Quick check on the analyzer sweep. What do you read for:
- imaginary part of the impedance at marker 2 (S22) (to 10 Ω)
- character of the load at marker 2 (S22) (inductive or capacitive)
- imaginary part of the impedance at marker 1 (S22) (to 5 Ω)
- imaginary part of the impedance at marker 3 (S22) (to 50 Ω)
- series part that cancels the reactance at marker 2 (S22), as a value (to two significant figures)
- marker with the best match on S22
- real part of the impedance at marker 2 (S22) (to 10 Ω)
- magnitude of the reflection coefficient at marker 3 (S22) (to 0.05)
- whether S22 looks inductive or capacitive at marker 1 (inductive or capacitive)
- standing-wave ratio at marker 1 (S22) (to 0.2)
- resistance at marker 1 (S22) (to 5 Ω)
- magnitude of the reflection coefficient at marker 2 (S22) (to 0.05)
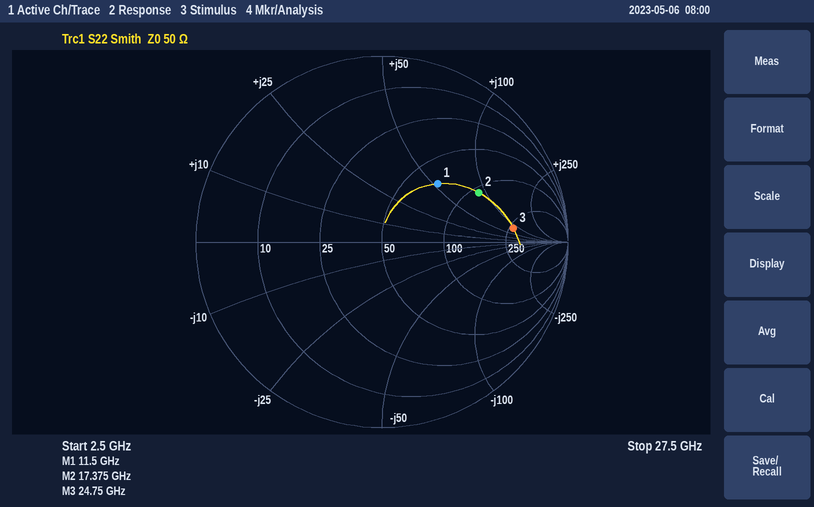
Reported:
+90 Ω
inductive
+55 Ω
+100 Ω
100 fF
marker 1
110 Ω
0.70
inductive
2.6
70 Ω
0.60
